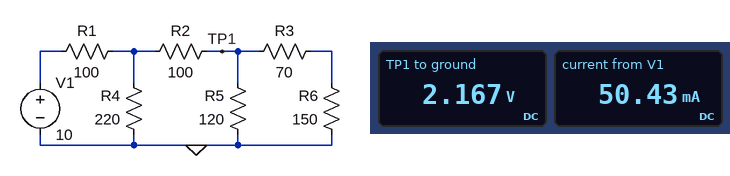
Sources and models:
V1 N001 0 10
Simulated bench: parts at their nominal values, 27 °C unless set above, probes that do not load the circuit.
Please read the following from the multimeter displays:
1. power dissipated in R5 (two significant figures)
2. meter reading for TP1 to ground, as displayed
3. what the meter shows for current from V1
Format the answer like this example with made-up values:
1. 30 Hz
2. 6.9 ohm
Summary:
1. 39 mW
2. 2.167 V
3. 50.43 mA
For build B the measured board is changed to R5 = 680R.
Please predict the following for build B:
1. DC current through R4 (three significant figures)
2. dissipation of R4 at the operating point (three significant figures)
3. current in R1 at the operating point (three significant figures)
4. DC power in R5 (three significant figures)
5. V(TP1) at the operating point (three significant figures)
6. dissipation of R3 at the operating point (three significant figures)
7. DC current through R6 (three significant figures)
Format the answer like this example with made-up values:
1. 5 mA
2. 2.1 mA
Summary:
1. 24.8 mA
2. 136 mW
3. 45.4 mA
4. 17.1 mW
5. 3.41 V
6. 16.8 mW
7. 15.5 mA
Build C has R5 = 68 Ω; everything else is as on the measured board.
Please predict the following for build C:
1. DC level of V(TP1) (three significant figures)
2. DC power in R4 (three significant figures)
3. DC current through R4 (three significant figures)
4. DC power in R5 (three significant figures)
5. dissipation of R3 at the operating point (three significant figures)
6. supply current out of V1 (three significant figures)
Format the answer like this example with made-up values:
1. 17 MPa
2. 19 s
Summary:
1. 1.62 V
2. 102 mW
3. 21.5 mA
4. 38.5 mW
5. 3.79 mW
6. 52.7 mA
